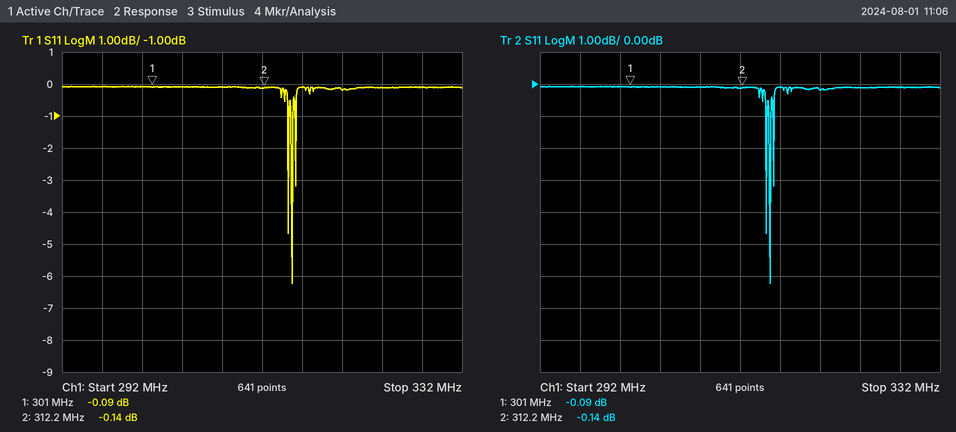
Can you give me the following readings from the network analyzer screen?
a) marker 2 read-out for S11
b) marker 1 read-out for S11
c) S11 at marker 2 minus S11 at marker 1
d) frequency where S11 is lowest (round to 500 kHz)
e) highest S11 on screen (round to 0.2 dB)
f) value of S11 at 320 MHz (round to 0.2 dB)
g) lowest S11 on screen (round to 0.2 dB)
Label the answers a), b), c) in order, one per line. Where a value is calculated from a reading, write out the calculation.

a) -0.14 dB
b) -0.09 dB
c) -0.14 − (-0.09) = -0.05 dB
d) 315.0 MHz
e) 0.0 dB
f) -0.2 dB
g) -6.2 dB
